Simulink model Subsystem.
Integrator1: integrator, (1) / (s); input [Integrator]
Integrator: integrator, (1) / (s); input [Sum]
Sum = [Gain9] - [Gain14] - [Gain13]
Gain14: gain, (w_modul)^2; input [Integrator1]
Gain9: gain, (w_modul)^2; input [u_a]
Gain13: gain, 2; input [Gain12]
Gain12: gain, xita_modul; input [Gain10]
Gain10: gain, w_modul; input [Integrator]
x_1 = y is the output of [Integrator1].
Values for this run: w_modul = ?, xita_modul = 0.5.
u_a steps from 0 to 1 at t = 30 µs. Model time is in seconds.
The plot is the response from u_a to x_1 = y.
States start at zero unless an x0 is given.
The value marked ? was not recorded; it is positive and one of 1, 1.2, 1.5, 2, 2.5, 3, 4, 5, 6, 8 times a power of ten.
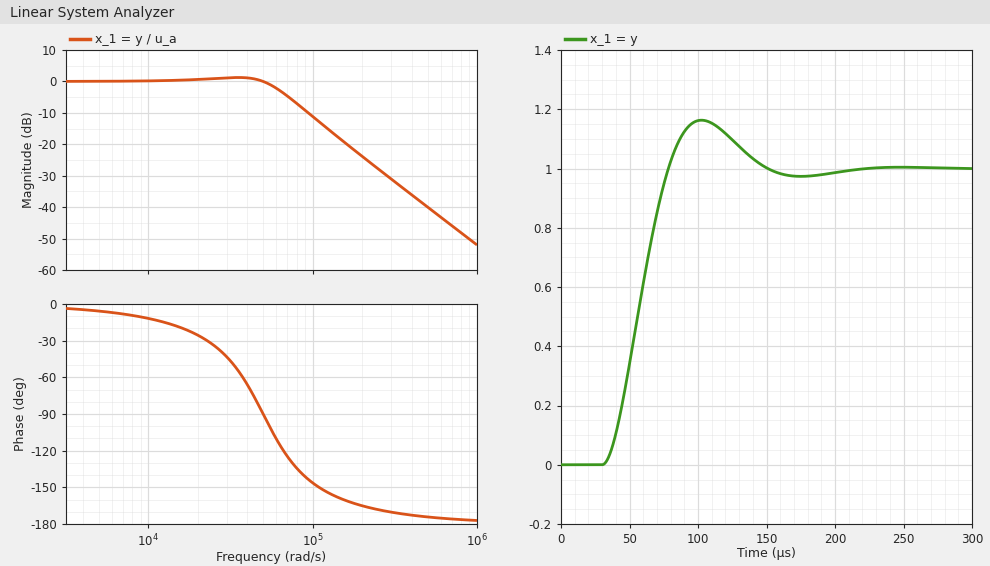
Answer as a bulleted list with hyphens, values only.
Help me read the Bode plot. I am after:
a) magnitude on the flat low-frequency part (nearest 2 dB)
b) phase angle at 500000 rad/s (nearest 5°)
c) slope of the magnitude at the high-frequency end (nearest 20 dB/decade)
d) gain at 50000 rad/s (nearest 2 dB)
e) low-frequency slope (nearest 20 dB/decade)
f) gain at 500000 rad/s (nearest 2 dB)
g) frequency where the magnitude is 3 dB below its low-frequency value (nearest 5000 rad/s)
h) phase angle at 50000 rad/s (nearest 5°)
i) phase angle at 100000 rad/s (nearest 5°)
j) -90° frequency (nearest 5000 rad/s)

- 0 dB
- -175°
- -40 dB/decade
- 0 dB
- 0 dB/decade
- -40 dB
- 65000 rad/s
- -90°
- -145°
- 50000 rad/s
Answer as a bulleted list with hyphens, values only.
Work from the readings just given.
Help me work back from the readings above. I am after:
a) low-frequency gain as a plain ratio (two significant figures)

- 1.0
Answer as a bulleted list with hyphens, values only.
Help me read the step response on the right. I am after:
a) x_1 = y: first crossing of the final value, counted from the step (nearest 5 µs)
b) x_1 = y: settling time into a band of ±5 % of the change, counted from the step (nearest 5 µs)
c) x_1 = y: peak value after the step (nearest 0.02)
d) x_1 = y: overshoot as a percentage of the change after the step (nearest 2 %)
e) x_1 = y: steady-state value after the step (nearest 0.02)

- 50 µs
- 105 µs
- 1.16
- 16 %
- 1.00
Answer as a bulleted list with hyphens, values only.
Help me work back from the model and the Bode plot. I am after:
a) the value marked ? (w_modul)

- 50000
